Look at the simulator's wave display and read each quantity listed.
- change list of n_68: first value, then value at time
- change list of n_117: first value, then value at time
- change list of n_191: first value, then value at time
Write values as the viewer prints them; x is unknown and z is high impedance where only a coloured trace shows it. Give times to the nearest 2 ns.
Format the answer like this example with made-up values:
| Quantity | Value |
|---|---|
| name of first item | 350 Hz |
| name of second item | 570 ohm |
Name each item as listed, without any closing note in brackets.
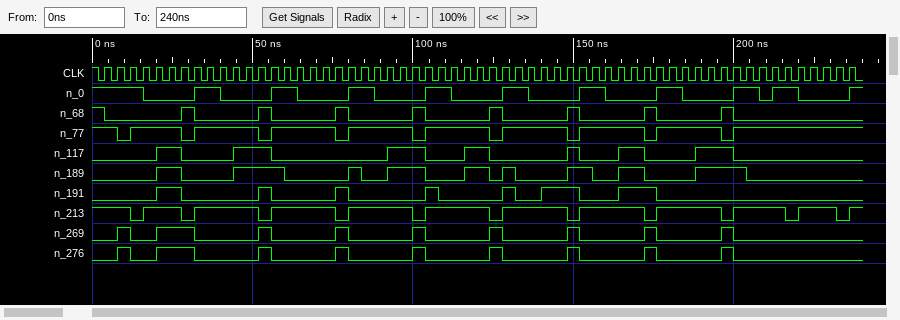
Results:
| Quantity | Value |
|---|---|
| change list of n_68: first value, then value at time | 1, 0 at 4 ns, 1 at 28 ns, 0 at 32 ns, 1 at 52 ns, 0 at 56 ns, 1 at 76 ns, 0 at 80 ns, 1 at 100 ns, 0 at 104 ns, 1 at 124 ns, 0 at 128 ns, 1 at 148 ns, 0 at 152 ns, 1 at 172 ns, 0 at 176 ns, 1 at 196 ns, 0 at 200 ns |
| change list of n_117: first value, then value at time | 0, 1 at 20 ns, 0 at 28 ns, 1 at 44 ns, 0 at 56 ns, 1 at 92 ns, 0 at 104 ns, 1 at 116 ns, 0 at 124 ns, 1 at 148 ns, 0 at 152 ns, 1 at 164 ns, 0 at 172 ns, 1 at 188 ns, 0 at 200 ns |
| change list of n_191: first value, then value at time | 0, 1 at 20 ns, 0 at 28 ns, 1 at 52 ns, 0 at 56 ns, 1 at 76 ns, 0 at 80 ns, 1 at 104 ns, 0 at 108 ns, 1 at 128 ns, 0 at 132 ns, 1 at 140 ns, 0 at 152 ns, 1 at 164 ns, 0 at 176 ns |
